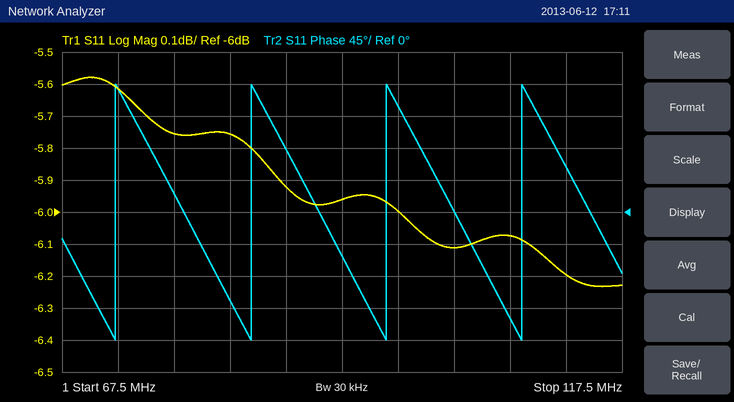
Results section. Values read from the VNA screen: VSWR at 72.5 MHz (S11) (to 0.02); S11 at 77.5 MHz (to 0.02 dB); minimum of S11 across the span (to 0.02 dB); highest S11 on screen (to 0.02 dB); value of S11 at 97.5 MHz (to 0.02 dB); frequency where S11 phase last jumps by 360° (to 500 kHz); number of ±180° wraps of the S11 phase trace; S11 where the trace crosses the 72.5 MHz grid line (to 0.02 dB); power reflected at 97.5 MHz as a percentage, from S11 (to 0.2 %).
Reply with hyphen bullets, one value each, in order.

- 3.20
- -5.76 dB
- -6.24 dB
- -5.58 dB
- -6.00 dB
- 108.5 MHz
- 4
- -5.62 dB
- 25.2 %
